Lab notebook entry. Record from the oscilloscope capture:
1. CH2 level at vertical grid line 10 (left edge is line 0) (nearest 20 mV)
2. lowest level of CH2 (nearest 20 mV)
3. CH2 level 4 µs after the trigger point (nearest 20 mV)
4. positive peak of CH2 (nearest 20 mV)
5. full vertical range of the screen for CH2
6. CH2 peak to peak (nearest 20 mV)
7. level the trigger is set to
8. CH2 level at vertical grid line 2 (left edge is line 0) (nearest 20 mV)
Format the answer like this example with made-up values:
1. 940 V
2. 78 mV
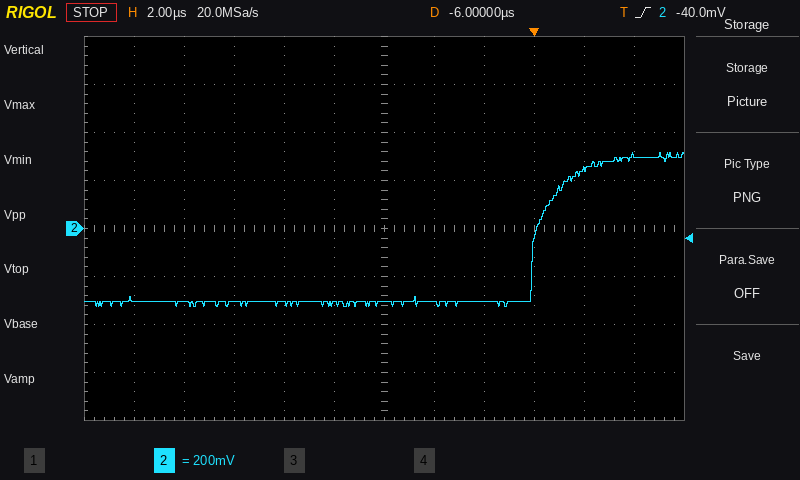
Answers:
1. 240 mV
2. -320 mV
3. 300 mV
4. 320 mV
5. 1.6 V
6. 640 mV
7. -40.0 mV
8. -300 mV
